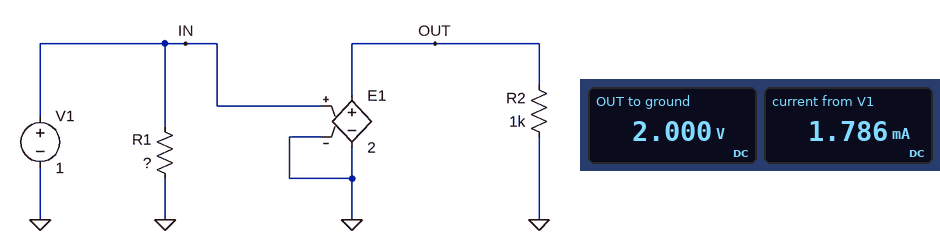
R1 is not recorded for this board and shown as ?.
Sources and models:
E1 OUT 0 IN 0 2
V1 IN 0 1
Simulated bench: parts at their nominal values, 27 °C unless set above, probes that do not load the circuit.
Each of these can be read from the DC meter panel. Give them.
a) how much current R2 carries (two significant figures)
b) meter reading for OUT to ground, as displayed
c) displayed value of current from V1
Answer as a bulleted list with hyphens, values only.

- 2.0 mA
- 2.000 V
- 1.786 mA
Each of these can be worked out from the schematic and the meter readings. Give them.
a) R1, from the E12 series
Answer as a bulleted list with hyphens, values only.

- 560 Ω
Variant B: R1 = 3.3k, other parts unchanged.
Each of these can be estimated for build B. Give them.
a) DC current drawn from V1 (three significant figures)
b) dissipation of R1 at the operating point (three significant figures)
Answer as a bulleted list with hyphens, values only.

- 303 µA
- 303 µW
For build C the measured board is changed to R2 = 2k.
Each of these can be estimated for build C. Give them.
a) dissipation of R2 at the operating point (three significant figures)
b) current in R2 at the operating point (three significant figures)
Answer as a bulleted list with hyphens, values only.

- 2.00 mW
- 1.00 mA
